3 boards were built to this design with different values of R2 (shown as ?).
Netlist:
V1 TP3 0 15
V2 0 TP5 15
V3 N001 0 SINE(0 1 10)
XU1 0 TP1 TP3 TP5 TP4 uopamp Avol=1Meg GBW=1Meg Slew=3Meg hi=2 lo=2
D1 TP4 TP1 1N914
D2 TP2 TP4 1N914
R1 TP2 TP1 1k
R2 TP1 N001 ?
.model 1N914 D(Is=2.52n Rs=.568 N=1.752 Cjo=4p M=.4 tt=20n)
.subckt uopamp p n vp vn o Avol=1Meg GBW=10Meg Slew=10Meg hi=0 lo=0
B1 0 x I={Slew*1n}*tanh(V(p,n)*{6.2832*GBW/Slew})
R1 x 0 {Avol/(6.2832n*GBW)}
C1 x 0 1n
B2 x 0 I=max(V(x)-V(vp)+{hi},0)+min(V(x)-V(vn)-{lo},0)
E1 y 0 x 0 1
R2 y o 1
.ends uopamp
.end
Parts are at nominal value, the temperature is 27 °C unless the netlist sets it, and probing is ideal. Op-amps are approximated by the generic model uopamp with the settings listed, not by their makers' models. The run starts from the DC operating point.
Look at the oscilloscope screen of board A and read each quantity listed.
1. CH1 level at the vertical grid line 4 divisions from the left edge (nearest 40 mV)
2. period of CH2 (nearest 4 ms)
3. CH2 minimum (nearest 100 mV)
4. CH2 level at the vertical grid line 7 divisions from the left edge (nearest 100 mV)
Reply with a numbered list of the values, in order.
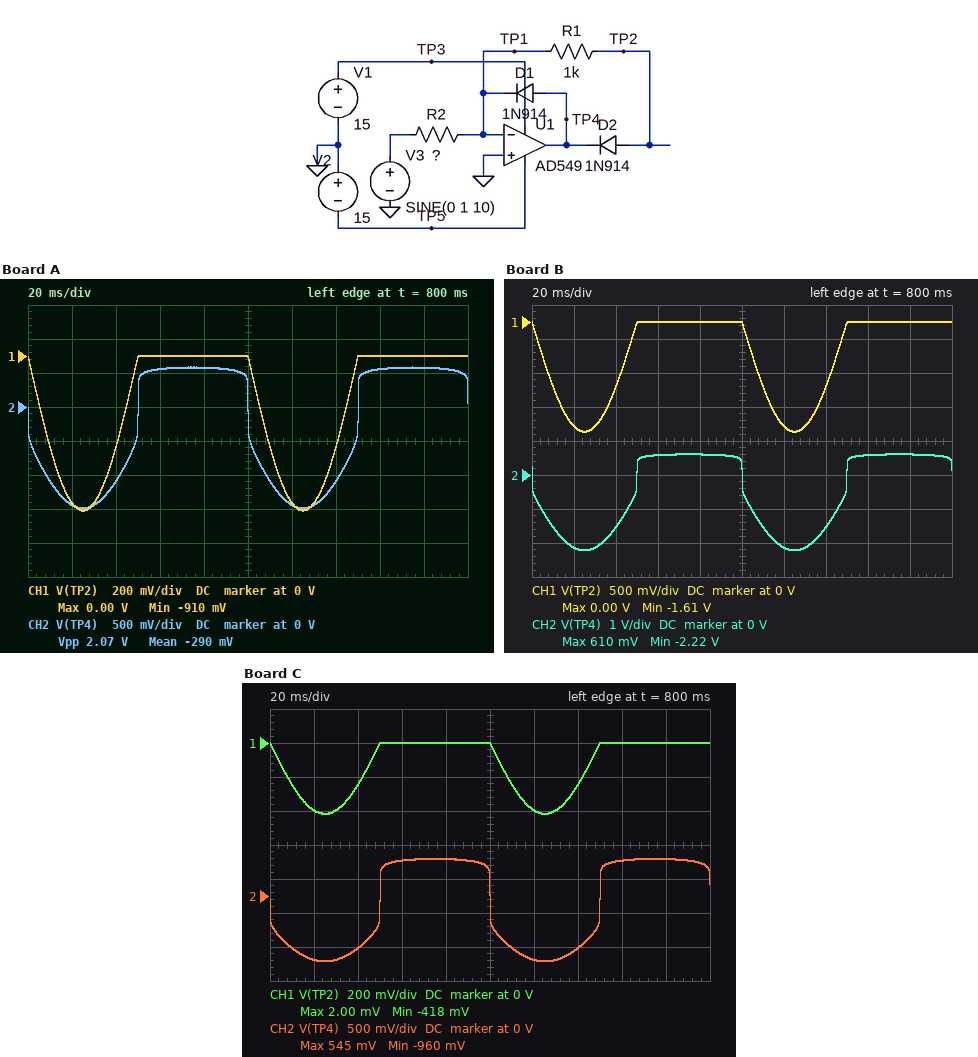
1. 0 V
2. 100 ms
3. -1.5 V
4. -1.1 V
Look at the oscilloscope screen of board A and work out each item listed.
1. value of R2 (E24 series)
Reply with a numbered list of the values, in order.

1. 1.1 kΩ
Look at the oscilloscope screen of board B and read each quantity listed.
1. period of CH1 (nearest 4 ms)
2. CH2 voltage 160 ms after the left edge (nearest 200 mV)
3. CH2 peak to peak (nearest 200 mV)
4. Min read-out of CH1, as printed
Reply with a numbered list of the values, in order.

1. 100 ms
2. 600 mV
3. 2.8 V
4. -1.61 V
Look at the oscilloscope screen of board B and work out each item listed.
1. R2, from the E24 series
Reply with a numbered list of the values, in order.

1. 620 Ω
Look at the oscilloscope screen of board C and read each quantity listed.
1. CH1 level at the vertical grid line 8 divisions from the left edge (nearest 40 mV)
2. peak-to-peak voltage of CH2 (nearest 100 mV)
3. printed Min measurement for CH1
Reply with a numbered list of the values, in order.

1. 0 V
2. 1.5 V
3. -418 mV
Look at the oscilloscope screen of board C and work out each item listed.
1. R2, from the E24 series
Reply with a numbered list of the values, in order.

1. 2.4 kΩ
